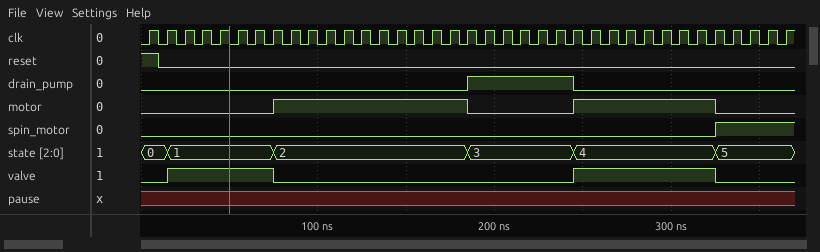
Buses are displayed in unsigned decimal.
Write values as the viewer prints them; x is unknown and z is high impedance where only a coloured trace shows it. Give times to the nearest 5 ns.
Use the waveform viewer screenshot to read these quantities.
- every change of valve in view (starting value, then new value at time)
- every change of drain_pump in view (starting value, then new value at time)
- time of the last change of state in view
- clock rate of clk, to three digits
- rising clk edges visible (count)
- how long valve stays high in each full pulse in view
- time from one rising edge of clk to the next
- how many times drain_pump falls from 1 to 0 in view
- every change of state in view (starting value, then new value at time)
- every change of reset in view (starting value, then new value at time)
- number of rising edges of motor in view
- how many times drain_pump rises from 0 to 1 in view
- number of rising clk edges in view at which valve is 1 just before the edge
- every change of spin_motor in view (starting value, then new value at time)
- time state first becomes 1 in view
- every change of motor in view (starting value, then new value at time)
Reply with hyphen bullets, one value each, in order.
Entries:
- 0, 1 at 15 ns, 0 at 75 ns, 1 at 245 ns, 0 at 325 ns
- 0, 1 at 185 ns, 0 at 245 ns
- 325 ns
- 100 MHz
- 37
- 60 ns, 80 ns
- 10 ns
- 1
- 0, 1 at 15 ns, 2 at 75 ns, 3 at 185 ns, 4 at 245 ns, 5 at 325 ns
- 1, 0 at 10 ns
- 2
- 1
- 14
- 0, 1 at 325 ns
- 15 ns
- 0, 1 at 75 ns, 0 at 185 ns, 1 at 245 ns, 0 at 325 ns
